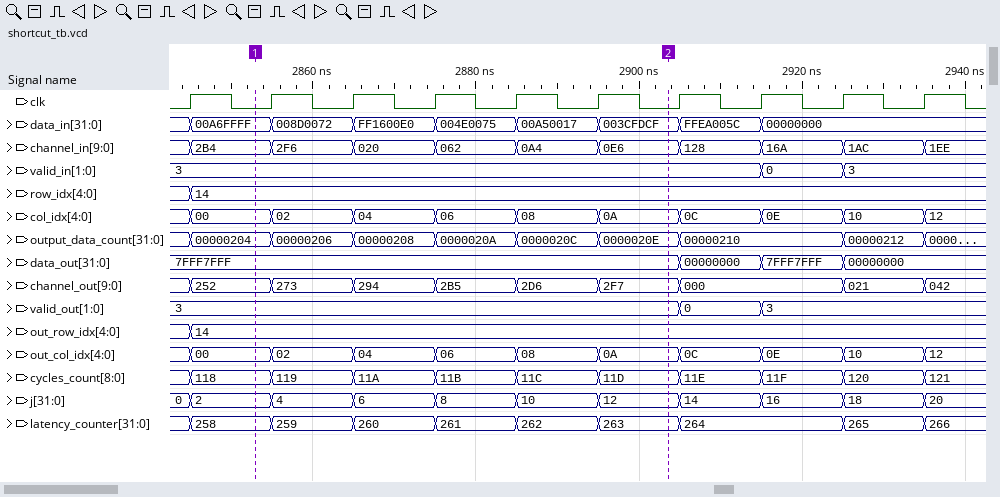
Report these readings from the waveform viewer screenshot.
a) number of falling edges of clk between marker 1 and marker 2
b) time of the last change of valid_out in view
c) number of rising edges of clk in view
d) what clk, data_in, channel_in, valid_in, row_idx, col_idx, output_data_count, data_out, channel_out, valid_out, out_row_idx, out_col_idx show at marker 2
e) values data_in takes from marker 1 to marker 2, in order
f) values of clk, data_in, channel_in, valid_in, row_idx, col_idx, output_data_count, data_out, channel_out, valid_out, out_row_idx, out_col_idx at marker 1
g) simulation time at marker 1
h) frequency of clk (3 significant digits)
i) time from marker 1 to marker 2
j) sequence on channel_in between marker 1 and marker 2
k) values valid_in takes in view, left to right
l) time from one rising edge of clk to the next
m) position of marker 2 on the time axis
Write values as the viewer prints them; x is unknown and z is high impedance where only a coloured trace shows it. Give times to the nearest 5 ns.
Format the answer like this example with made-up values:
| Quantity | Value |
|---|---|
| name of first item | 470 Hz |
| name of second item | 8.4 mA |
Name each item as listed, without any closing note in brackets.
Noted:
| Quantity | Value |
|---|---|
| number of falling edges of clk between marker 1 and marker 2 | 5 |
| time of the last change of valid_out in view | 2915 ns |
| number of rising edges of clk in view | 10 |
| what clk, data_in, channel_in, valid_in, row_idx, col_idx, output_data_count, data_out, channel_out, valid_out, out_row_idx, out_col_idx show at marker 2 | clk=0, data_in=003CFDCF, channel_in=0E6, valid_in=3, row_idx=14, col_idx=0A, output_data_count=0000020E, data_out=7FFF7FFF, channel_out=2F7, valid_out=3, out_row_idx=14, out_col_idx=0A |
| values data_in takes from marker 1 to marker 2, in order | 00A6FFFF, 008D0072, FF1600E0, 004E0075, 00A50017, 003CFDCF |
| values of clk, data_in, channel_in, valid_in, row_idx, col_idx, output_data_count, data_out, channel_out, valid_out, out_row_idx, out_col_idx at marker 1 | clk=0, data_in=00A6FFFF, channel_in=2B4, valid_in=3, row_idx=14, col_idx=00, output_data_count=00000204, data_out=7FFF7FFF, channel_out=252, valid_out=3, out_row_idx=14, out_col_idx=00 |
| simulation time at marker 1 | 2855 ns |
| frequency of clk | 100 MHz |
| time from marker 1 to marker 2 | 50 ns |
| sequence on channel_in between marker 1 and marker 2 | 2B4, 2F6, 020, 062, 0A4, 0E6 |
| values valid_in takes in view, left to right | 3, 0, 3 |
| time from one rising edge of clk to the next | 10 ns |
| position of marker 2 on the time axis | 2905 ns |
